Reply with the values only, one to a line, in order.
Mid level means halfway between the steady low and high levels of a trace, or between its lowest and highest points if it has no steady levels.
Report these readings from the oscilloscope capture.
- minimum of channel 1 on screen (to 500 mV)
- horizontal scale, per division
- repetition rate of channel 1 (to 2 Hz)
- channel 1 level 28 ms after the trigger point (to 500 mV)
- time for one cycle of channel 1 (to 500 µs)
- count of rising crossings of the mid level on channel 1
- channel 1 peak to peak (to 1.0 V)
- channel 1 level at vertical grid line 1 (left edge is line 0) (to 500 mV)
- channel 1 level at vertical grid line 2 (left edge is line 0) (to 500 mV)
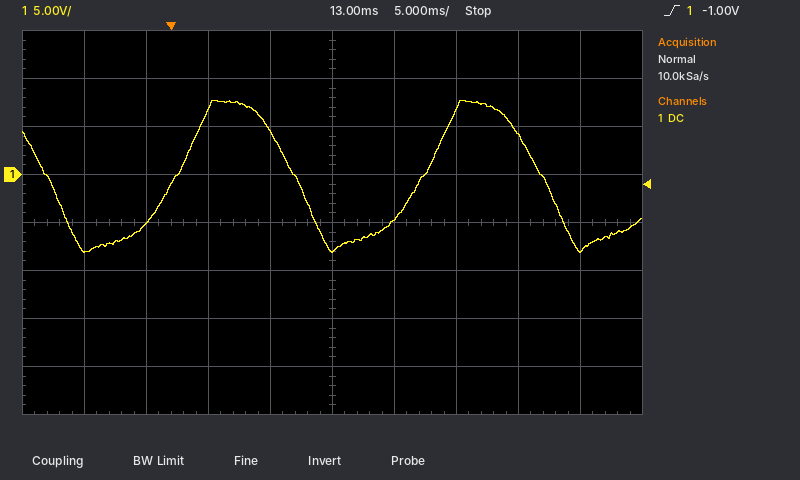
-8.0 V
5 ms
50 Hz
4.0 V
20.0 ms
2
16.0 V
-8.0 V
-5.0 V
